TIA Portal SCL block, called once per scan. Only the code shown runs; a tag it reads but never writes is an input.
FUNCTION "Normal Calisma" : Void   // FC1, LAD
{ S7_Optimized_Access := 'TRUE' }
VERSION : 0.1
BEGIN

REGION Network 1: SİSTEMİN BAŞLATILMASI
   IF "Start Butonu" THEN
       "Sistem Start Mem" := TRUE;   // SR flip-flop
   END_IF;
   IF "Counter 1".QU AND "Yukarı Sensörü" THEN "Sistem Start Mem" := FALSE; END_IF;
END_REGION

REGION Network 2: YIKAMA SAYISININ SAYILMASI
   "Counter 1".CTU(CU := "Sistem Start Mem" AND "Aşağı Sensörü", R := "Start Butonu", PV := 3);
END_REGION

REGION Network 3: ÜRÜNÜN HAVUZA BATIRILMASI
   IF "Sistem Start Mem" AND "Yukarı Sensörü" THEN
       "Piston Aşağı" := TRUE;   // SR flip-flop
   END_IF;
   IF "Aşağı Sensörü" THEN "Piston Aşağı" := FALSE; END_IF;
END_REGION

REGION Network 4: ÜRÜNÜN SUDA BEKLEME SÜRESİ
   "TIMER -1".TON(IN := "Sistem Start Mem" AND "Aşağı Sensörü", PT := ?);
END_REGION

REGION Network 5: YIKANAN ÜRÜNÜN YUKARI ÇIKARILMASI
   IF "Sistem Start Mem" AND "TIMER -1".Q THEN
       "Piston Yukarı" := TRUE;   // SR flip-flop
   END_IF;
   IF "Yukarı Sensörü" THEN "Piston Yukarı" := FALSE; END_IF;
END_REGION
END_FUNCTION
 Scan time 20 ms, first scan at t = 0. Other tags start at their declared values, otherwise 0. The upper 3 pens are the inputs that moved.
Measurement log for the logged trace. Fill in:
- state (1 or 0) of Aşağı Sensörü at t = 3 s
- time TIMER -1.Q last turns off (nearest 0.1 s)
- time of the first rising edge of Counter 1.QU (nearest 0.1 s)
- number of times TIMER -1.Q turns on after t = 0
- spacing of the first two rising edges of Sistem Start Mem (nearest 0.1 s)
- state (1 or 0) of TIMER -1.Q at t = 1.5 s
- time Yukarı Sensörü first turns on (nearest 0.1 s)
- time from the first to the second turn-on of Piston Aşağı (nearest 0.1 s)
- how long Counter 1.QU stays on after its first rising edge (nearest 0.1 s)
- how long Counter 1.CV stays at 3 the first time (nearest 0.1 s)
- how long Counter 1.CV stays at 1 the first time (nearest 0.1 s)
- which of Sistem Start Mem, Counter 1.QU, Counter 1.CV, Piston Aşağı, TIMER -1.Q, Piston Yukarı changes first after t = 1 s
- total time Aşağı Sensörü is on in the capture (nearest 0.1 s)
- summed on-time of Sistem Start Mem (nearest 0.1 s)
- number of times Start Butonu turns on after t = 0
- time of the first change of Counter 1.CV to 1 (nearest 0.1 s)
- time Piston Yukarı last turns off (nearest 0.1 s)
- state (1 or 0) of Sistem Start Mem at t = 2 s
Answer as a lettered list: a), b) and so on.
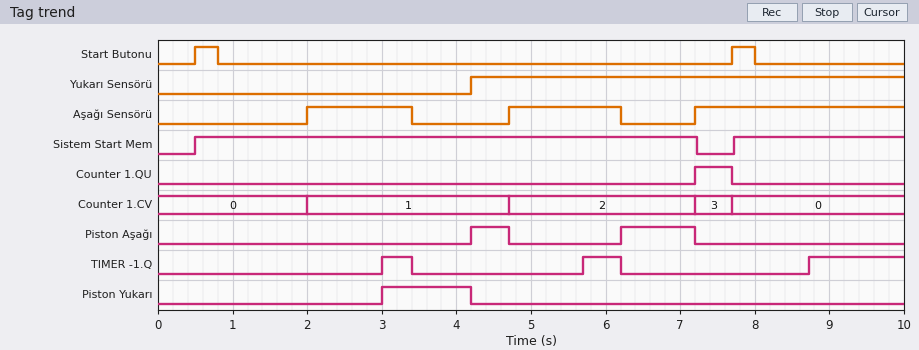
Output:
a) 1
b) 6.2 s
c) 7.2 s
d) 3
e) 7.2 s
f) 0
g) 4.2 s
h) 2.0 s
i) 0.5 s
j) 0.5 s
k) 2.7 s
l) Counter 1.CV
m) 5.7 s
n) 9.0 s
o) 2
p) 2.0 s
q) 4.2 s
r) 1
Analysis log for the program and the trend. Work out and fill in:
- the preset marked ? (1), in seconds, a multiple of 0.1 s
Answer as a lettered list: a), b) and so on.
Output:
a) 1.0 s
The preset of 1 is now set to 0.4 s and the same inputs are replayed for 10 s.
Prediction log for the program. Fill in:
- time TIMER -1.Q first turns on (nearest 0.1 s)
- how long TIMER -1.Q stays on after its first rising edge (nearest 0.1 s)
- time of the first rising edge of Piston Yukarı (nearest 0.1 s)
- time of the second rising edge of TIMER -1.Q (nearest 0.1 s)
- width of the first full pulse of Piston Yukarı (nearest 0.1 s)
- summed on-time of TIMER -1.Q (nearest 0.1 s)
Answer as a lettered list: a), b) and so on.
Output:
a) 2.4 s
b) 1.0 s
c) 2.4 s
d) 5.1 s
e) 1.8 s
f) 4.0 s
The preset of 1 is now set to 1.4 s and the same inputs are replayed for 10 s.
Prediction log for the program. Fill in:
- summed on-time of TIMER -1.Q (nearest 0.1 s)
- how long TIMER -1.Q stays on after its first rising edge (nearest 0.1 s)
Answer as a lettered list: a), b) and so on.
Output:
a) 1.0 s
b) 0.1 s
